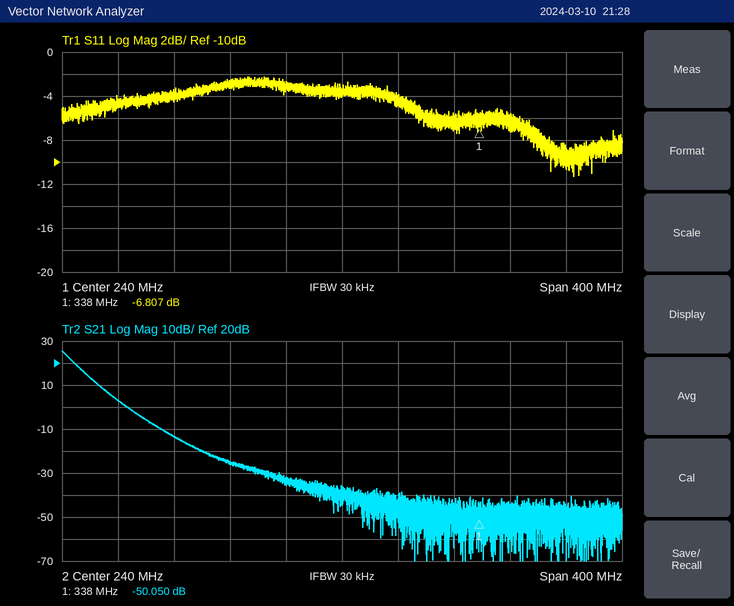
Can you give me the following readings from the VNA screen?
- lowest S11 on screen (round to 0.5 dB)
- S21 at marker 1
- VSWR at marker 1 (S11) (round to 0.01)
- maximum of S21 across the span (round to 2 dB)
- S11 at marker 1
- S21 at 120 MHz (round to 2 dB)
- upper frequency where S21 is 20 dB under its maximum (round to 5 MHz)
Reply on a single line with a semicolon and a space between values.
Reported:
-11.5 dB; -50.050 dB; 2.68; 26 dB; -6.807 dB; -14 dB; 75 MHz
